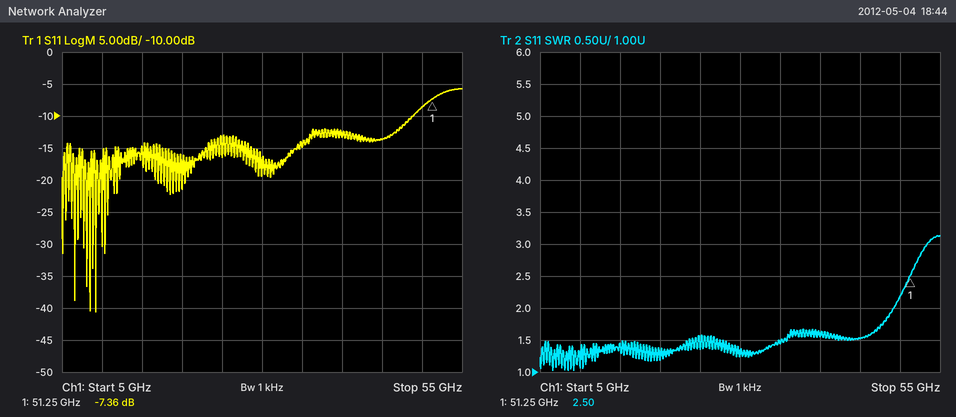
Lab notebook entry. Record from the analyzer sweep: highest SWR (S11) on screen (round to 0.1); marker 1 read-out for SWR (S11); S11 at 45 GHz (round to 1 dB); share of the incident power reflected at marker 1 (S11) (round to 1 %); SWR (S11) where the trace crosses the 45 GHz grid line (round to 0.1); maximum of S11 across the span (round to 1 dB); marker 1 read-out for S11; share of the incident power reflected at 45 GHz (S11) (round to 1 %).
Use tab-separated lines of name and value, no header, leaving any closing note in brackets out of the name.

highest SWR (S11) on screen	3.1
marker 1 read-out for SWR	2.50
S11 at 45 GHz	-14 dB
share of the incident power reflected at marker 1 (S11)	18 %
SWR (S11) where the trace crosses the 45 GHz grid line	1.5
maximum of S11 across the span	-6 dB
marker 1 read-out for S11	-7.36 dB
share of the incident power reflected at 45 GHz (S11)	4 %
